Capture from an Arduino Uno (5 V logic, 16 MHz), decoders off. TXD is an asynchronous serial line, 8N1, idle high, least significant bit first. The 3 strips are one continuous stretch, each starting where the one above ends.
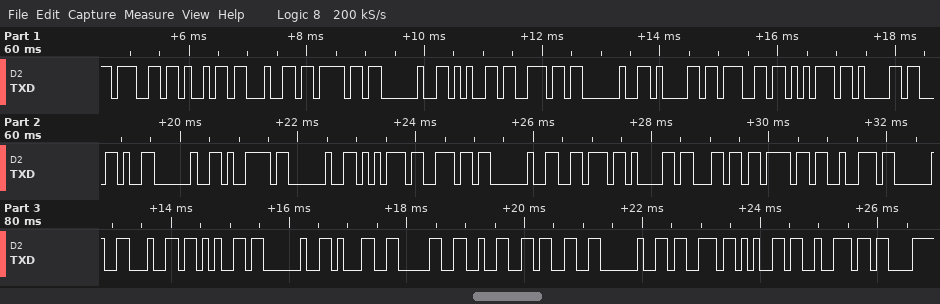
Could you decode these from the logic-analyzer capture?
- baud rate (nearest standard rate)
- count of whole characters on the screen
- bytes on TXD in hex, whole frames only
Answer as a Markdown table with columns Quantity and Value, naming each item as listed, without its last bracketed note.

| Quantity | Value |
|---|---|
| baud rate | 9600 baud |
| count of whole characters on the screen | 37 |
| bytes on TXD in hex, whole frames only | 0x67 0x69 0x64 0x6F 0x20 0x65 0x6E 0x20 0x61 0x67 0x75 0x61 0x2C 0x20 0x79 0x20 0x75 0x6E 0x20 0x76 0x61 0x6C 0x6F 0x72 0x20 0x64 0x65 0x20 0x31 0x30 0x32 0x33 0x20 0x73 0x65 0x72 0xC3 |
